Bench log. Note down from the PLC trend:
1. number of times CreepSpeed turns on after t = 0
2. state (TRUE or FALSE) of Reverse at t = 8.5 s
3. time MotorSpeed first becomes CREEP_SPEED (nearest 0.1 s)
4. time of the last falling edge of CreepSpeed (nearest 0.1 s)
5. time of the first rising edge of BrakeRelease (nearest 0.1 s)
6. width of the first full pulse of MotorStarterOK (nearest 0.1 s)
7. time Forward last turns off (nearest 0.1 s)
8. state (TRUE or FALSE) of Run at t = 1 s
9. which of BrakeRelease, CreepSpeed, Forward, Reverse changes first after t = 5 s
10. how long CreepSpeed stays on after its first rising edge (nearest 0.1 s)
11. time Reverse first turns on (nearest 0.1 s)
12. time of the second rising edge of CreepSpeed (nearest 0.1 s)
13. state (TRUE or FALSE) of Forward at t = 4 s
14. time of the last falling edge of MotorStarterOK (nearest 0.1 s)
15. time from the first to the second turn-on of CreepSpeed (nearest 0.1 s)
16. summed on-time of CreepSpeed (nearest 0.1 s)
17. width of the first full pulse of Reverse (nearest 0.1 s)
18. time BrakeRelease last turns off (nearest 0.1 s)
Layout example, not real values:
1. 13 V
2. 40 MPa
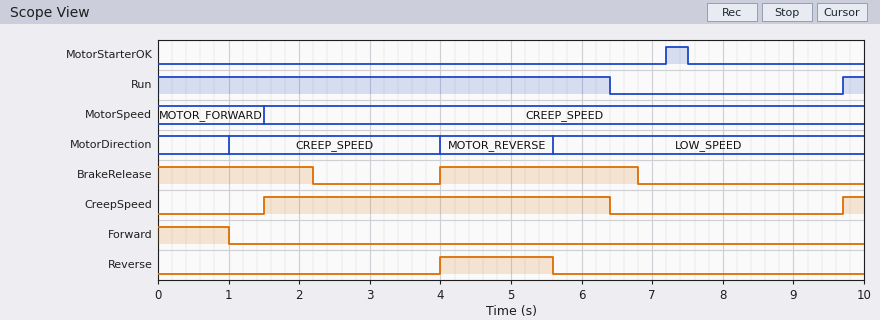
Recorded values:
1. 2
2. FALSE
3. 1.5 s
4. 6.4 s
5. 4.0 s
6. 0.3 s
7. 1.0 s
8. TRUE
9. Reverse
10. 4.9 s
11. 4.0 s
12. 9.7 s
13. FALSE
14. 7.5 s
15. 8.2 s
16. 5.2 s
17. 1.6 s
18. 6.8 s
